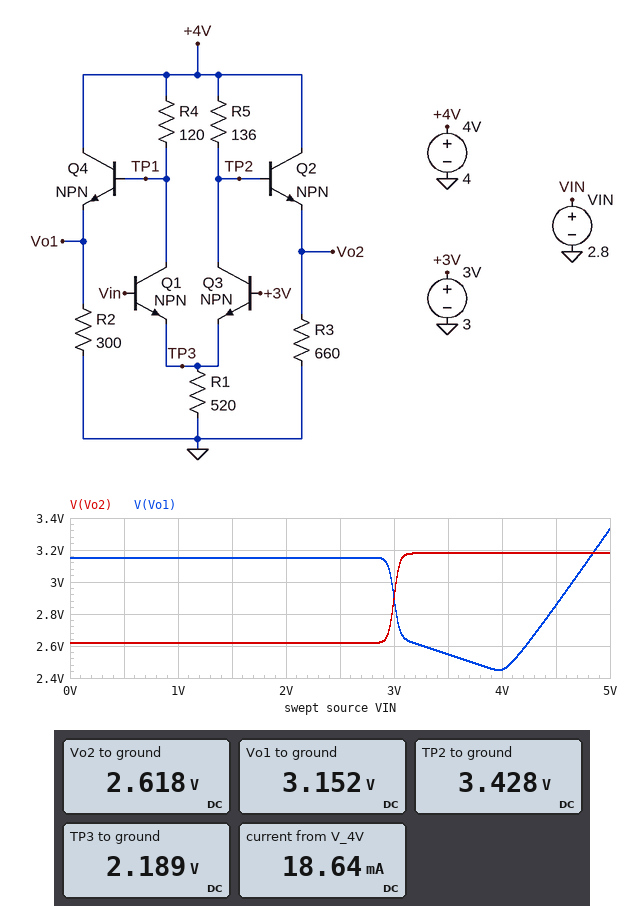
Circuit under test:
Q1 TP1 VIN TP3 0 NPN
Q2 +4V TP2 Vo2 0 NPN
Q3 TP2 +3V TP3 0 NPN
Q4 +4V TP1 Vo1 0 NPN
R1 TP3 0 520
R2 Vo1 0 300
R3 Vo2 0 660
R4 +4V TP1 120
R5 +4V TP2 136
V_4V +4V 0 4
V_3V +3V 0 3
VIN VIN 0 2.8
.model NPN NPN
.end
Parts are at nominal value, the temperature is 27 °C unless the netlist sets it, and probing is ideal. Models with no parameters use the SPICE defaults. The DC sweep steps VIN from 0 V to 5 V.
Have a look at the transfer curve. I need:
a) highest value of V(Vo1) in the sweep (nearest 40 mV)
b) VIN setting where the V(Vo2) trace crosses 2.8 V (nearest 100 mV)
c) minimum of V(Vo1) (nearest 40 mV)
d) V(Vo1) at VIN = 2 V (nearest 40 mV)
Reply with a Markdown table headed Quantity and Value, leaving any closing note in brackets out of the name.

| Quantity | Value |
|---|---|
| highest value of V(Vo1) in the sweep | 3.32 V |
| VIN setting where the V(Vo2) trace crosses 2.8 V | 3.0 V |
| minimum of V(Vo1) | 2.44 V |
| V(Vo1) at VIN = 2 V | 3.16 V |
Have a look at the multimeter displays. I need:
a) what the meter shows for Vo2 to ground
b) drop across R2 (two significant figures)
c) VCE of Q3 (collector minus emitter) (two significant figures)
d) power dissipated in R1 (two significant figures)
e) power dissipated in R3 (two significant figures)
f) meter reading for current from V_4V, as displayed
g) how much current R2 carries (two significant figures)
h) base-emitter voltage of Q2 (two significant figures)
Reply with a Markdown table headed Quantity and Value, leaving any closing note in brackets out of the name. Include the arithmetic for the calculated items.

| Quantity | Value |
|---|---|
| what the meter shows for Vo2 to ground | 2.618 V |
| drop across R2 | 3.152 V = 3.2 V |
| VCE of Q3 (collector minus emitter) | 3.428 V - 2.189 V = 1.2 V |
| power dissipated in R1 | (2.189 V)^2 / 520 Ω = 9.2 mW |
| power dissipated in R3 | (2.618 V)^2 / 660 Ω = 10 mW |
| meter reading for current from V_4V, as displayed | 18.64 mA |
| how much current R2 carries | (3.152 V) / 300 Ω = 11 mA |
| base-emitter voltage of Q2 | 3.428 V - 2.618 V = 810 mV |
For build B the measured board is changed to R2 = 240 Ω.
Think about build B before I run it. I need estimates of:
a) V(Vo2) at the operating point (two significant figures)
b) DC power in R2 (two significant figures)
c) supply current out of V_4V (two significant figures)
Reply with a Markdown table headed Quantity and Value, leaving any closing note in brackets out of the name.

| Quantity | Value |
|---|---|
| V(Vo2) at the operating point | 2.6 V |
| DC power in R2 | 41 mW |
| supply current out of V_4V | 21 mA |
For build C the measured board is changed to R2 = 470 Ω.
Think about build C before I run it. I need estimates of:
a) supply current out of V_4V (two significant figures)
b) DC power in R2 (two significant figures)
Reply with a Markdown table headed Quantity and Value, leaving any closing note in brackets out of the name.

| Quantity | Value |
|---|---|
| supply current out of V_4V | 15 mA |
| DC power in R2 | 21 mW |
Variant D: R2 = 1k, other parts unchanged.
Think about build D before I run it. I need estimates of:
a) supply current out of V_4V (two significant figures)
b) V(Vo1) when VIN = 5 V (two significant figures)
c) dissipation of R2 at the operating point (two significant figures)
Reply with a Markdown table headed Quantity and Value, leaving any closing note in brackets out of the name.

| Quantity | Value |
|---|---|
| supply current out of V_4V | 11 mA |
| V(Vo1) when VIN = 5 V | 3.4 V |
| dissipation of R2 at the operating point | 10 mW |
